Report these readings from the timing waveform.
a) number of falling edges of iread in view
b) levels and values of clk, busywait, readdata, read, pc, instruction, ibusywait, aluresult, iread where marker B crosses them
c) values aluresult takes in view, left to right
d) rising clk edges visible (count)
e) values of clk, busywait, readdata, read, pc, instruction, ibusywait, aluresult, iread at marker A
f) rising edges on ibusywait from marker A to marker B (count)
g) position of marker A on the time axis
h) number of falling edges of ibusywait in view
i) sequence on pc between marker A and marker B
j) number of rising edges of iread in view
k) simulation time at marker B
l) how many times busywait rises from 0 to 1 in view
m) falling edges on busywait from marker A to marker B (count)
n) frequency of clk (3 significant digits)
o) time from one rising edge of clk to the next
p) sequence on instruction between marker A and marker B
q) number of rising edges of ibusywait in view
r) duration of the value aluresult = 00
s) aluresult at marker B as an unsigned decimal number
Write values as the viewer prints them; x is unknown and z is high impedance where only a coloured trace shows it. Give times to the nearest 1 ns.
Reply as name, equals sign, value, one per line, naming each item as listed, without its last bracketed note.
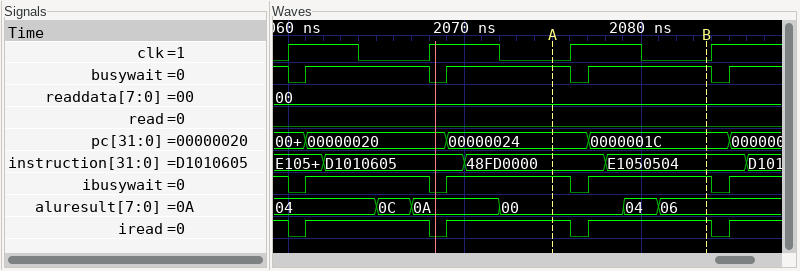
number of falling edges of iread in view = 4
levels and values of clk, busywait, readdata, read, pc, instruction, ibusywait, aluresult, iread where marker B crosses them = clk=0, busywait=1, readdata=00, read=0, pc=0000001C, instruction=E1050504, ibusywait=1, aluresult=06, iread=1
values aluresult takes in view, left to right = 04, 0C, 0A, 00, 04, 06
rising clk edges visible = 4
values of clk, busywait, readdata, read, pc, instruction, ibusywait, aluresult, iread at marker A = clk=0, busywait=1, readdata=00, read=0, pc=00000024, instruction=48FD0000, ibusywait=1, aluresult=00, iread=1
rising edges on ibusywait from marker A to marker B = 1
position of marker A on the time axis = 2075 ns
number of falling edges of ibusywait in view = 4
sequence on pc between marker A and marker B = 00000024, 0000001C
number of rising edges of iread in view = 4
simulation time at marker B = 2084 ns
how many times busywait rises from 0 to 1 in view = 4
falling edges on busywait from marker A to marker B = 1
frequency of clk = 125 MHz
time from one rising edge of clk to the next = 8 ns
sequence on instruction between marker A and marker B = 48FD0000, E1050504
number of rising edges of ibusywait in view = 4
duration of the value aluresult = 00 = 7 ns
aluresult at marker B as an unsigned decimal number = 6
